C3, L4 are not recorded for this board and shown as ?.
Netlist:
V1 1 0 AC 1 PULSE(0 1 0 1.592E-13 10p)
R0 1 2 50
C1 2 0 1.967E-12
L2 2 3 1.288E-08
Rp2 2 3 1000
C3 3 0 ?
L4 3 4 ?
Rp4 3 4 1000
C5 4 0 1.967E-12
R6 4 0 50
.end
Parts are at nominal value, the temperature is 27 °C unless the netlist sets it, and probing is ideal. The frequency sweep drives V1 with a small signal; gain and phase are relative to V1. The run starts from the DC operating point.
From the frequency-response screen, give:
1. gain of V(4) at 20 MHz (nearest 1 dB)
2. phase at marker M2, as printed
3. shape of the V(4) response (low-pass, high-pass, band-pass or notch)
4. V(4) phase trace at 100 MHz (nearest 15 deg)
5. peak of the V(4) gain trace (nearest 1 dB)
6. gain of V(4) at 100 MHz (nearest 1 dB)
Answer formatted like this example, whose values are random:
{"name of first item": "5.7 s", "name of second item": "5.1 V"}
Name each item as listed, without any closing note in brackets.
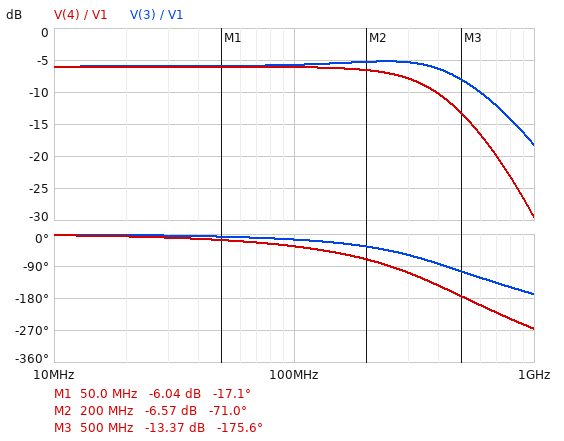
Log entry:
{"gain of V(4) at 20 MHz": "-6 dB", "phase at marker M2, as printed": "-71.0 deg", "shape of the V(4) response": "low-pass", "V(4) phase trace at 100 MHz": "-30 deg", "peak of the V(4) gain trace": "-6 dB", "gain of V(4) at 100 MHz": "-6 dB"}
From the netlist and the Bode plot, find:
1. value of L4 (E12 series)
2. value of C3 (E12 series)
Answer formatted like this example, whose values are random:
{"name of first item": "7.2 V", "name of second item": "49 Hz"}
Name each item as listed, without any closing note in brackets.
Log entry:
{"value of L4": "27 nH", "value of C3": "18 pF"}
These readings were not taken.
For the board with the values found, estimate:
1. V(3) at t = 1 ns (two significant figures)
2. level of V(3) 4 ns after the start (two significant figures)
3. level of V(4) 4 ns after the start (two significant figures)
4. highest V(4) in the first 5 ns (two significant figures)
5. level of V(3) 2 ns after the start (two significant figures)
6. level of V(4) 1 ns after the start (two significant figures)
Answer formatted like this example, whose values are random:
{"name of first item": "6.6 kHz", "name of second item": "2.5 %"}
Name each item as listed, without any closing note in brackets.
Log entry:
{"V(3) at t = 1 ns": "520 mV", "level of V(3) 4 ns after the start": "500 mV", "level of V(4) 4 ns after the start": "500 mV", "highest V(4) in the first 5 ns": "520 mV", "level of V(3) 2 ns after the start": "530 mV", "level of V(4) 1 ns after the start": "270 mV"}
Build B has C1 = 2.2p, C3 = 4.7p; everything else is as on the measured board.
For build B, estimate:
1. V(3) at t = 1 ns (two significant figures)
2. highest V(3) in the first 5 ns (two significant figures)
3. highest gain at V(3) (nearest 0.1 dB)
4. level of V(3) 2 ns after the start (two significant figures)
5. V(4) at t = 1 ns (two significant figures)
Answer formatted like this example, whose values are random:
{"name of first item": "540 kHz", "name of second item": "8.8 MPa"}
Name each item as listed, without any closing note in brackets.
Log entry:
{"V(3) at t = 1 ns": "550 mV", "highest V(3) in the first 5 ns": "750 mV", "highest gain at V(3)": "-0.8 dB", "level of V(3) 2 ns after the start": "510 mV", "V(4) at t = 1 ns": "490 mV"}
